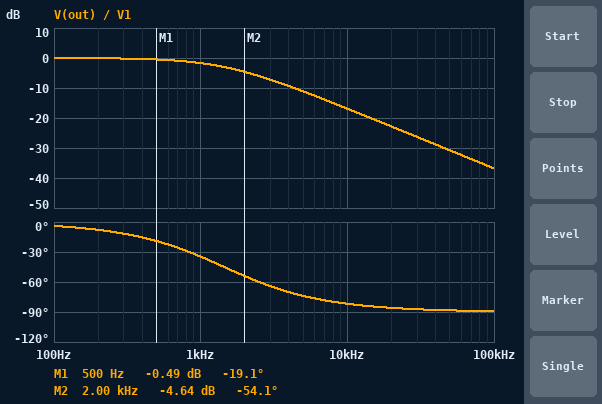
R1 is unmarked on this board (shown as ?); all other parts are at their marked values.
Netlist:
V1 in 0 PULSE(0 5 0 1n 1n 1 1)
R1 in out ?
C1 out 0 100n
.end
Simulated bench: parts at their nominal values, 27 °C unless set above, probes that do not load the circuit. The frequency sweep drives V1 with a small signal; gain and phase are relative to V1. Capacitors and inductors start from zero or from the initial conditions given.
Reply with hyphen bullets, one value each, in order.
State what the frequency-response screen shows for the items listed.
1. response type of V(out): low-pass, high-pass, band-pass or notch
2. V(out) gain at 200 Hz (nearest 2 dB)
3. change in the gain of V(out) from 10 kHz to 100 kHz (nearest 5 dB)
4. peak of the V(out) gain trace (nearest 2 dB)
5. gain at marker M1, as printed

- low-pass
- 0 dB
- -20 dB
- 0 dB
- -0.49 dB
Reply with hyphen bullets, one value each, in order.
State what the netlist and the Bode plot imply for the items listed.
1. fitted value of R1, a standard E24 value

- 1.1 kΩ
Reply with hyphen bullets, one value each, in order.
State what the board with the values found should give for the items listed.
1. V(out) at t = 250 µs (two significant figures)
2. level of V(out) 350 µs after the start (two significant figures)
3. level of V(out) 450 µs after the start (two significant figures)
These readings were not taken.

- 4.5 V
- 4.8 V
- 4.9 V
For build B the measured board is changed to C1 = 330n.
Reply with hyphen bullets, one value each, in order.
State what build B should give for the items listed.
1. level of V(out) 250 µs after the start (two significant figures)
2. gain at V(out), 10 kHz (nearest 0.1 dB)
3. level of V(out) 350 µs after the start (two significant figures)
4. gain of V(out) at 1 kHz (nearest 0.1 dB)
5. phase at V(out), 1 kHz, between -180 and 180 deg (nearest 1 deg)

- 2.5 V
- -27.2 dB
- 3.1 V
- -7.9 dB
- -66 deg
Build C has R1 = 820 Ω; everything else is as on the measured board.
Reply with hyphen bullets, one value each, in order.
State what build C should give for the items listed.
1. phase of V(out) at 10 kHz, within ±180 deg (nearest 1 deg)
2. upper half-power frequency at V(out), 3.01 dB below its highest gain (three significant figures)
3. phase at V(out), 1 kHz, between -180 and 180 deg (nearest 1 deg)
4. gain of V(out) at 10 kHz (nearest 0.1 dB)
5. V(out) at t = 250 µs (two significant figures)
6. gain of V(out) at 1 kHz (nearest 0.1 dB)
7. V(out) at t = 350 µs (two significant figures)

- -79 deg
- 1.94 kHz
- -27 deg
- -14.4 dB
- 4.8 V
- -1.0 dB
- 4.9 V
